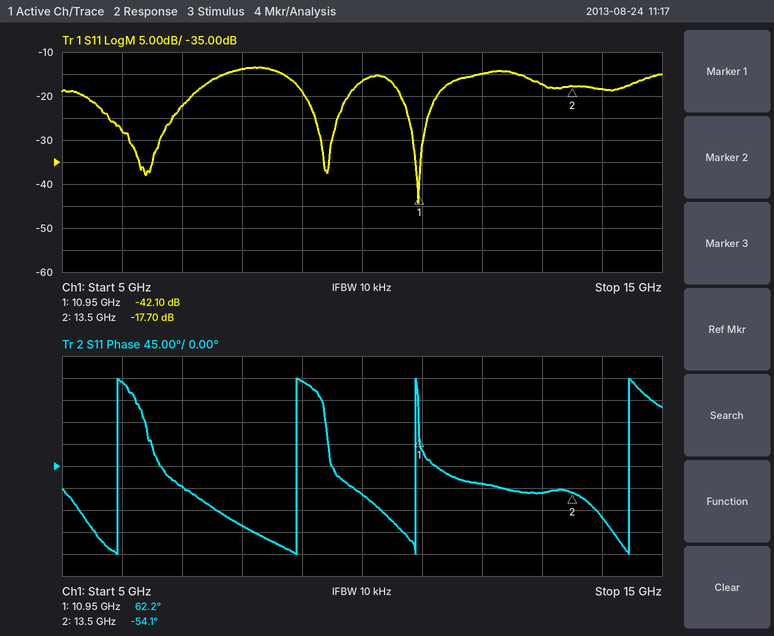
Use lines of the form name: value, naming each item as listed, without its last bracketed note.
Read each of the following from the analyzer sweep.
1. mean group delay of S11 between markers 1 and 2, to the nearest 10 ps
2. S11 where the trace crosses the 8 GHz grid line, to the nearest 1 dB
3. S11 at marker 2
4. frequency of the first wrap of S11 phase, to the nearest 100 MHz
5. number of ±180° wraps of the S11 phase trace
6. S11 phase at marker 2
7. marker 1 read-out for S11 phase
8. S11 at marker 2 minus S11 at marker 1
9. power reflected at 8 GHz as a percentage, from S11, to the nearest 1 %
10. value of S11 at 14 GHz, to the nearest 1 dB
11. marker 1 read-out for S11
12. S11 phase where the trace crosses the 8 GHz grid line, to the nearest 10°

mean group delay of S11 between markers 1 and 2, to the nearest 10 ps: 130 ps
S11 where the trace crosses the 8 GHz grid line, to the nearest 1 dB: -14 dB
S11 at marker 2: -17.70 dB
frequency of the first wrap of S11 phase, to the nearest 100 MHz: 5.9 GHz
number of ±180° wraps of the S11 phase trace: 4
S11 phase at marker 2: -54.1°
marker 1 read-out for S11 phase: 62.2°
S11 at marker 2 minus S11 at marker 1: 24.40 dB
power reflected at 8 GHz as a percentage, from S11, to the nearest 1 %: 4 %
value of S11 at 14 GHz, to the nearest 1 dB: -18 dB
marker 1 read-out for S11: -42.10 dB
S11 phase where the trace crosses the 8 GHz grid line, to the nearest 10°: -120°
